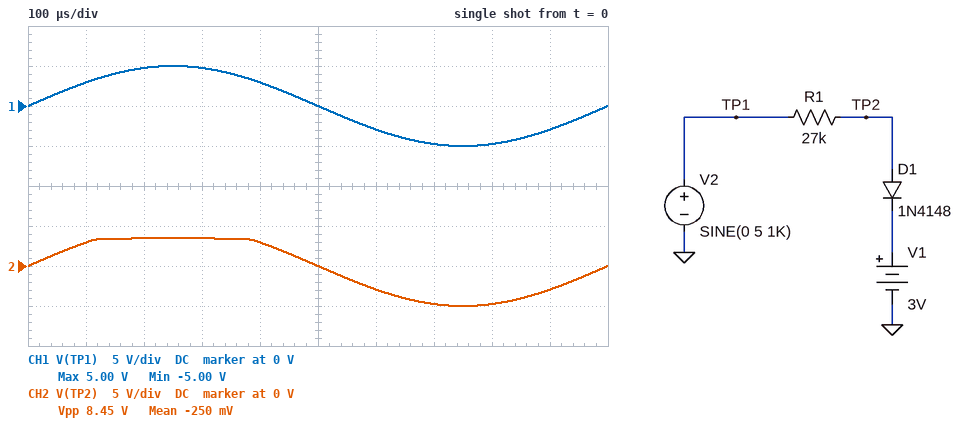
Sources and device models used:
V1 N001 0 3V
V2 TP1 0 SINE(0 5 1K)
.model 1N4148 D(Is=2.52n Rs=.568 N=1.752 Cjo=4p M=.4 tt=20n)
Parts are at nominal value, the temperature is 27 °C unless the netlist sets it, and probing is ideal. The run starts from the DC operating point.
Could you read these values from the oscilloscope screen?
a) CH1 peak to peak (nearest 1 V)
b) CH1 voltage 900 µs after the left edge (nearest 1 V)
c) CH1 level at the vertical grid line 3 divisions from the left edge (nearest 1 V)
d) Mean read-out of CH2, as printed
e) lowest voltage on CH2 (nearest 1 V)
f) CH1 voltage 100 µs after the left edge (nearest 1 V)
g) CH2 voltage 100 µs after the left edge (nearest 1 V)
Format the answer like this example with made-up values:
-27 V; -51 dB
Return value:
10 V; -3 V; 5 V; -250 mV; -5 V; 3 V; 3 V
